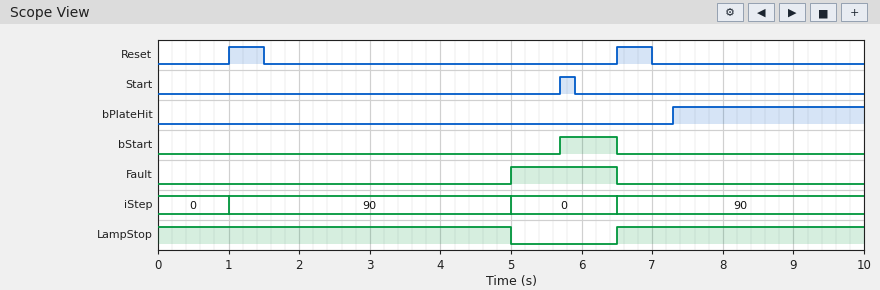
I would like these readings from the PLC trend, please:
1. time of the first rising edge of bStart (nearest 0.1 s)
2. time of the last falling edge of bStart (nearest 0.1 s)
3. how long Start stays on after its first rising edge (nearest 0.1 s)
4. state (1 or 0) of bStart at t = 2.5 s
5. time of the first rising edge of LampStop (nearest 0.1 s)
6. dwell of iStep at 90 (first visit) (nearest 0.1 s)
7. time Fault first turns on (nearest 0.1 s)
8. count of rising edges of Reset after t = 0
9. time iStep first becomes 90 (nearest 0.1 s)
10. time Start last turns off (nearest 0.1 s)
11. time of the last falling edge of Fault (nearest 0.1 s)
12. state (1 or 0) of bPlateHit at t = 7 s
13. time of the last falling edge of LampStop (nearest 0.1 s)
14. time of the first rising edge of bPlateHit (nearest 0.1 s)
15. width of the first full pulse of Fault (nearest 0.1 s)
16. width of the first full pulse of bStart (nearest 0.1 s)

5.7 s
6.5 s
0.2 s
0
6.5 s
4.0 s
5.0 s
2
1.0 s
5.9 s
6.5 s
0
5.0 s
7.3 s
1.5 s
0.8 s
